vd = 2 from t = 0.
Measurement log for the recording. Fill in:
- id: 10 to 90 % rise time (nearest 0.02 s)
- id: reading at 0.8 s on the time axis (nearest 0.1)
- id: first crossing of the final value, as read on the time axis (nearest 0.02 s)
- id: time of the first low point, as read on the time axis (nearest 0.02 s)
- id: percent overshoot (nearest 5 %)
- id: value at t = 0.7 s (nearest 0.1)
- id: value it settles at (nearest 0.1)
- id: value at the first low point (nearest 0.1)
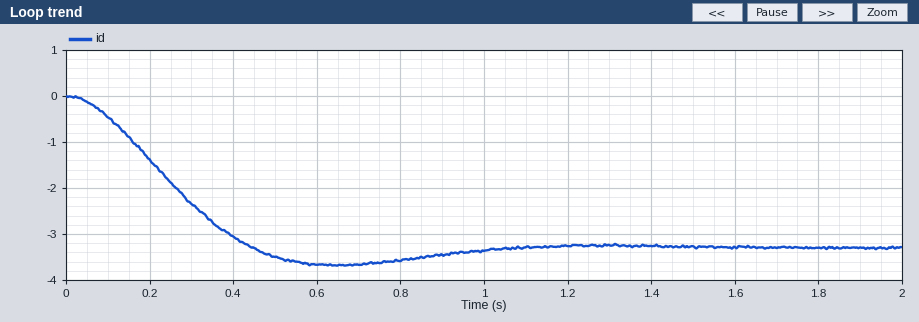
0.30 s
-3.6
0.44 s
0.64 s
10 %
-3.7
-3.3
-3.7
